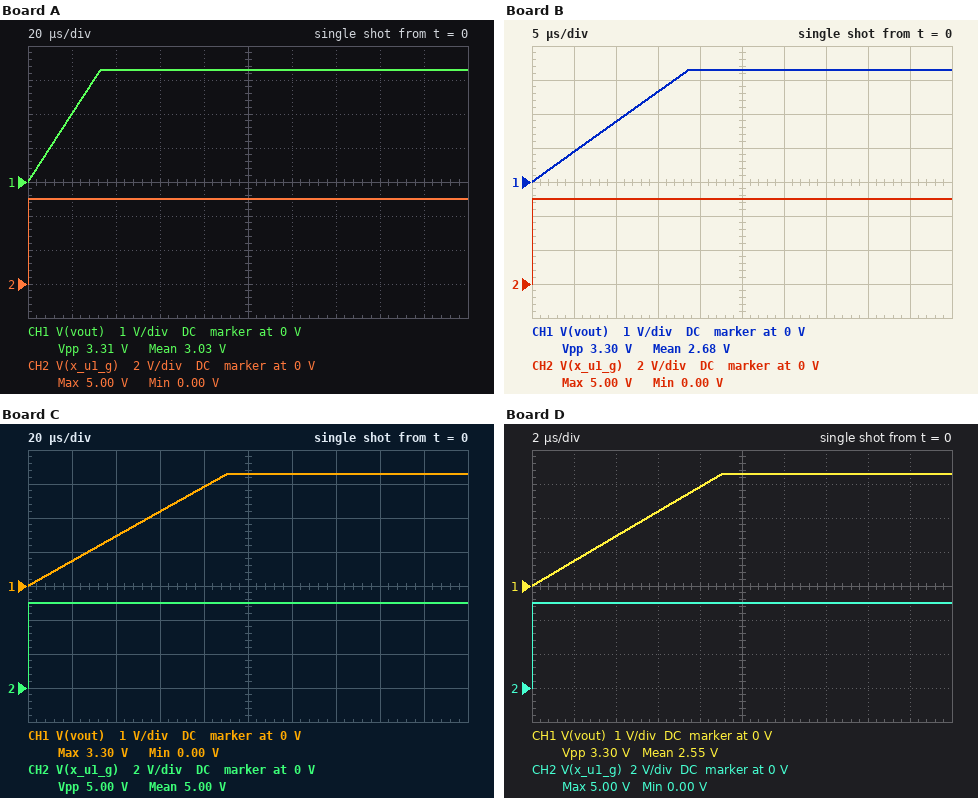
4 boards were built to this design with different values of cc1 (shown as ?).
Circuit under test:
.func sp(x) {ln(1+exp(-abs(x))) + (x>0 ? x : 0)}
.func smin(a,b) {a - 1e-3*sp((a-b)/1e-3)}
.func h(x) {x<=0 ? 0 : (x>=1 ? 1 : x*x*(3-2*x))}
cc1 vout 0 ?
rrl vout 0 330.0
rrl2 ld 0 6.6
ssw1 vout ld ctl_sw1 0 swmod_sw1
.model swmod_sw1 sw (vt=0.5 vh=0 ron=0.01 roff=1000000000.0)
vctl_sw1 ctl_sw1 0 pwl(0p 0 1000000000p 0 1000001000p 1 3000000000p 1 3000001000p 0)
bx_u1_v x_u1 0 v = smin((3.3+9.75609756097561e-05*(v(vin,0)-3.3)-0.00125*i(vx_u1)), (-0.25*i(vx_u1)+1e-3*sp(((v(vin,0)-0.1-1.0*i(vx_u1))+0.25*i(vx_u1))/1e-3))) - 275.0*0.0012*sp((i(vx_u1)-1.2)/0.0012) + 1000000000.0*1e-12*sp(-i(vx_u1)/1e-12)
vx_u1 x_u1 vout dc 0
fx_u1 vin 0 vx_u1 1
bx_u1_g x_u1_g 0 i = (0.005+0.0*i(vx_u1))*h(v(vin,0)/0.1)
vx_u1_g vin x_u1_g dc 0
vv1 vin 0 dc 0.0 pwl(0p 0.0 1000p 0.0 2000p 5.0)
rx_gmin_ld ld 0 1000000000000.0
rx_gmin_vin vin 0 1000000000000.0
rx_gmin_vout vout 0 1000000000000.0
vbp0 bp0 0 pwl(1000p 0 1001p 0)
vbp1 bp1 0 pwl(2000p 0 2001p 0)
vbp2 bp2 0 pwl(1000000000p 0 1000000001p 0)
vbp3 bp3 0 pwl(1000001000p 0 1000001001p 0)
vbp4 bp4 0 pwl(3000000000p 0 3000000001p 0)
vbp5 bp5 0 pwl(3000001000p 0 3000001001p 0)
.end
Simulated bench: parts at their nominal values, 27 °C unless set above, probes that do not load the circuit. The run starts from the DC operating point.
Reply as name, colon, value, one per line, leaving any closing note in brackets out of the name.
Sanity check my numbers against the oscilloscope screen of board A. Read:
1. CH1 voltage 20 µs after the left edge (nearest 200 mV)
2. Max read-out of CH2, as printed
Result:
CH1 voltage 20 µs after the left edge: 2.0 V
Max read-out of CH2, as printed: 5.00 V
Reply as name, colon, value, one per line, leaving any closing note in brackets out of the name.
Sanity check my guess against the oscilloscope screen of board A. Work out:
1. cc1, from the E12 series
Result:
cc1, from the E12 series: 12 µF
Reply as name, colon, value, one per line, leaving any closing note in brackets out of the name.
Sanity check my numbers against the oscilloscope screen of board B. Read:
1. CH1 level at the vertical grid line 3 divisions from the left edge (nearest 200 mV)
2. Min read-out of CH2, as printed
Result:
CH1 level at the vertical grid line 3 divisions from the left edge: 2.6 V
Min read-out of CH2, as printed: 0.00 V
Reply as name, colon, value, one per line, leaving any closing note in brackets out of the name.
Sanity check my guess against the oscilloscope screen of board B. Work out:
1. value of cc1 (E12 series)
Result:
value of cc1: 6.8 µF
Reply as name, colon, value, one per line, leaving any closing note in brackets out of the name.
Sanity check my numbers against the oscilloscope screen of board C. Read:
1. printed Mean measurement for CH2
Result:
printed Mean measurement for CH2: 5.00 V
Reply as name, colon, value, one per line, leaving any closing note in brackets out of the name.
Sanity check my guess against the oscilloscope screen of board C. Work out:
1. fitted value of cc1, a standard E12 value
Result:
fitted value of cc1, a standard E12 value: 33 µF
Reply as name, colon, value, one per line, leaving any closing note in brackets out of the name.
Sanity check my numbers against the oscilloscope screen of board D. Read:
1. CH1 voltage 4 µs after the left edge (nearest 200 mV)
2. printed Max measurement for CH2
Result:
CH1 voltage 4 µs after the left edge: 1.4 V
printed Max measurement for CH2: 5.00 V
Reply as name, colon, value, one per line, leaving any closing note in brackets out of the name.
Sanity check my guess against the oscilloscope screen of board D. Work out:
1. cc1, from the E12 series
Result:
cc1, from the E12 series: 3.3 µF
